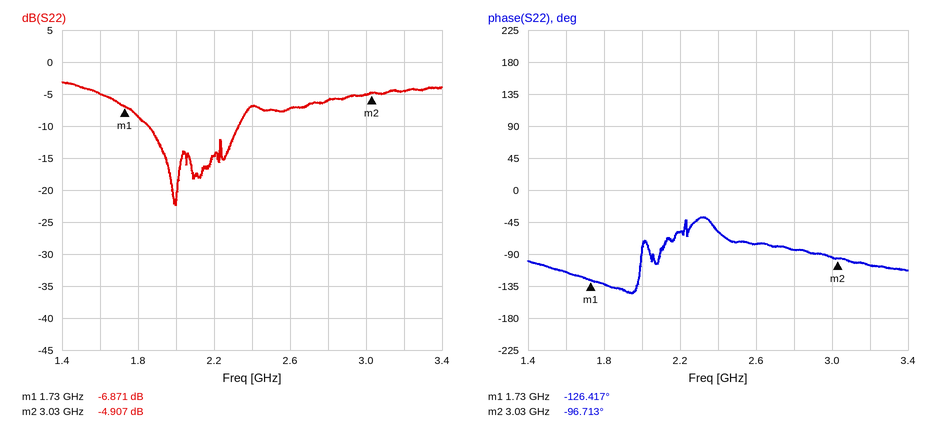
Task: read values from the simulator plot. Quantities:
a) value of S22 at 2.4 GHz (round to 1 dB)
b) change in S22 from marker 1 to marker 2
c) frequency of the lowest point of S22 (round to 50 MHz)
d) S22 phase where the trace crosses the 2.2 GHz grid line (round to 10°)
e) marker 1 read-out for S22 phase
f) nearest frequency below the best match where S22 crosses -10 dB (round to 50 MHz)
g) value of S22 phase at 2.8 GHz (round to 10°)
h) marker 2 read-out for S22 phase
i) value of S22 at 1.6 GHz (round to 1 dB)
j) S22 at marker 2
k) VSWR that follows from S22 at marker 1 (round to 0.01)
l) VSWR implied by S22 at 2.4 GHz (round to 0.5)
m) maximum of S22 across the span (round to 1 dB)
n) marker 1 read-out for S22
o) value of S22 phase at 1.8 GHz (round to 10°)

-7 dB
1.964 dB
2.00 GHz
-60°
-126.417°
1.85 GHz
-80°
-96.713°
-5 dB
-4.907 dB
2.66
2.5
-3 dB
-6.871 dB
-130°
